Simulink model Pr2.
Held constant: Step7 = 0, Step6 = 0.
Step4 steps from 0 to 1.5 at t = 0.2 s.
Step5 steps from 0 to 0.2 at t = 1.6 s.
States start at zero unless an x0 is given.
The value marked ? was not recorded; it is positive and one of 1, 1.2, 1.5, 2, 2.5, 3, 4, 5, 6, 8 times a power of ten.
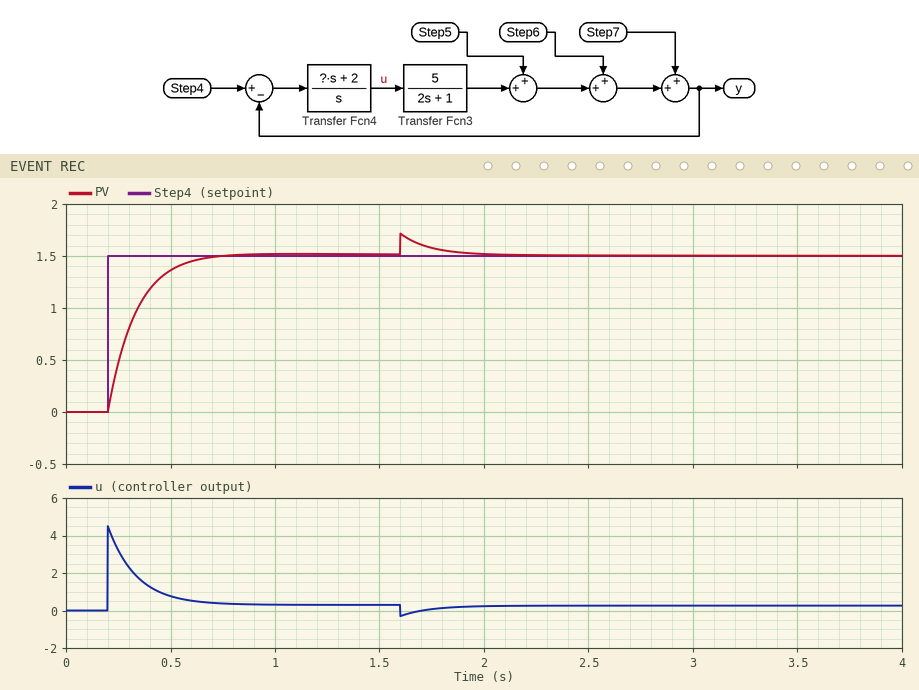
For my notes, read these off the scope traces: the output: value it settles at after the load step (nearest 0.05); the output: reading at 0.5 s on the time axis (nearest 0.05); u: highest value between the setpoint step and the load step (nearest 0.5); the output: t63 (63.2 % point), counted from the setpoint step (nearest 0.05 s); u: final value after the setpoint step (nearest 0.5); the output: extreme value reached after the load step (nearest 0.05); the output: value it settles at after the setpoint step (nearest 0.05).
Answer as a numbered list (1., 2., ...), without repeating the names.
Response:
1. 1.50
2. 1.35
3. 4.5
4. 0.15 s
5. 0.5
6. 1.70
7. 1.50
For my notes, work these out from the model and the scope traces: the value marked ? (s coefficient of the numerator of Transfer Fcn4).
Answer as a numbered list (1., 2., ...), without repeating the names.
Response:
1. 3
